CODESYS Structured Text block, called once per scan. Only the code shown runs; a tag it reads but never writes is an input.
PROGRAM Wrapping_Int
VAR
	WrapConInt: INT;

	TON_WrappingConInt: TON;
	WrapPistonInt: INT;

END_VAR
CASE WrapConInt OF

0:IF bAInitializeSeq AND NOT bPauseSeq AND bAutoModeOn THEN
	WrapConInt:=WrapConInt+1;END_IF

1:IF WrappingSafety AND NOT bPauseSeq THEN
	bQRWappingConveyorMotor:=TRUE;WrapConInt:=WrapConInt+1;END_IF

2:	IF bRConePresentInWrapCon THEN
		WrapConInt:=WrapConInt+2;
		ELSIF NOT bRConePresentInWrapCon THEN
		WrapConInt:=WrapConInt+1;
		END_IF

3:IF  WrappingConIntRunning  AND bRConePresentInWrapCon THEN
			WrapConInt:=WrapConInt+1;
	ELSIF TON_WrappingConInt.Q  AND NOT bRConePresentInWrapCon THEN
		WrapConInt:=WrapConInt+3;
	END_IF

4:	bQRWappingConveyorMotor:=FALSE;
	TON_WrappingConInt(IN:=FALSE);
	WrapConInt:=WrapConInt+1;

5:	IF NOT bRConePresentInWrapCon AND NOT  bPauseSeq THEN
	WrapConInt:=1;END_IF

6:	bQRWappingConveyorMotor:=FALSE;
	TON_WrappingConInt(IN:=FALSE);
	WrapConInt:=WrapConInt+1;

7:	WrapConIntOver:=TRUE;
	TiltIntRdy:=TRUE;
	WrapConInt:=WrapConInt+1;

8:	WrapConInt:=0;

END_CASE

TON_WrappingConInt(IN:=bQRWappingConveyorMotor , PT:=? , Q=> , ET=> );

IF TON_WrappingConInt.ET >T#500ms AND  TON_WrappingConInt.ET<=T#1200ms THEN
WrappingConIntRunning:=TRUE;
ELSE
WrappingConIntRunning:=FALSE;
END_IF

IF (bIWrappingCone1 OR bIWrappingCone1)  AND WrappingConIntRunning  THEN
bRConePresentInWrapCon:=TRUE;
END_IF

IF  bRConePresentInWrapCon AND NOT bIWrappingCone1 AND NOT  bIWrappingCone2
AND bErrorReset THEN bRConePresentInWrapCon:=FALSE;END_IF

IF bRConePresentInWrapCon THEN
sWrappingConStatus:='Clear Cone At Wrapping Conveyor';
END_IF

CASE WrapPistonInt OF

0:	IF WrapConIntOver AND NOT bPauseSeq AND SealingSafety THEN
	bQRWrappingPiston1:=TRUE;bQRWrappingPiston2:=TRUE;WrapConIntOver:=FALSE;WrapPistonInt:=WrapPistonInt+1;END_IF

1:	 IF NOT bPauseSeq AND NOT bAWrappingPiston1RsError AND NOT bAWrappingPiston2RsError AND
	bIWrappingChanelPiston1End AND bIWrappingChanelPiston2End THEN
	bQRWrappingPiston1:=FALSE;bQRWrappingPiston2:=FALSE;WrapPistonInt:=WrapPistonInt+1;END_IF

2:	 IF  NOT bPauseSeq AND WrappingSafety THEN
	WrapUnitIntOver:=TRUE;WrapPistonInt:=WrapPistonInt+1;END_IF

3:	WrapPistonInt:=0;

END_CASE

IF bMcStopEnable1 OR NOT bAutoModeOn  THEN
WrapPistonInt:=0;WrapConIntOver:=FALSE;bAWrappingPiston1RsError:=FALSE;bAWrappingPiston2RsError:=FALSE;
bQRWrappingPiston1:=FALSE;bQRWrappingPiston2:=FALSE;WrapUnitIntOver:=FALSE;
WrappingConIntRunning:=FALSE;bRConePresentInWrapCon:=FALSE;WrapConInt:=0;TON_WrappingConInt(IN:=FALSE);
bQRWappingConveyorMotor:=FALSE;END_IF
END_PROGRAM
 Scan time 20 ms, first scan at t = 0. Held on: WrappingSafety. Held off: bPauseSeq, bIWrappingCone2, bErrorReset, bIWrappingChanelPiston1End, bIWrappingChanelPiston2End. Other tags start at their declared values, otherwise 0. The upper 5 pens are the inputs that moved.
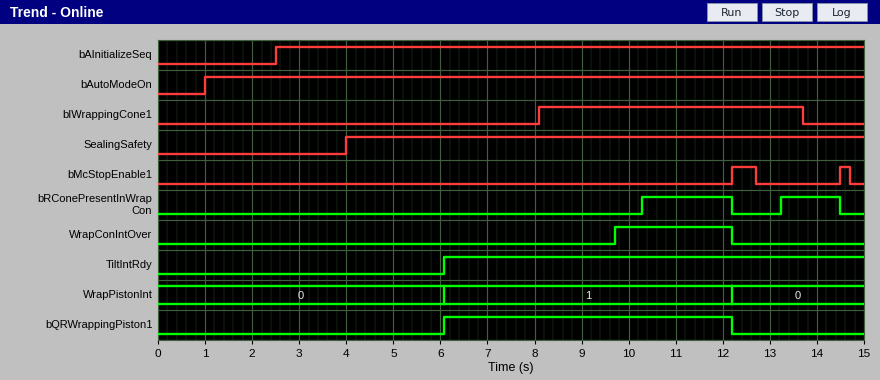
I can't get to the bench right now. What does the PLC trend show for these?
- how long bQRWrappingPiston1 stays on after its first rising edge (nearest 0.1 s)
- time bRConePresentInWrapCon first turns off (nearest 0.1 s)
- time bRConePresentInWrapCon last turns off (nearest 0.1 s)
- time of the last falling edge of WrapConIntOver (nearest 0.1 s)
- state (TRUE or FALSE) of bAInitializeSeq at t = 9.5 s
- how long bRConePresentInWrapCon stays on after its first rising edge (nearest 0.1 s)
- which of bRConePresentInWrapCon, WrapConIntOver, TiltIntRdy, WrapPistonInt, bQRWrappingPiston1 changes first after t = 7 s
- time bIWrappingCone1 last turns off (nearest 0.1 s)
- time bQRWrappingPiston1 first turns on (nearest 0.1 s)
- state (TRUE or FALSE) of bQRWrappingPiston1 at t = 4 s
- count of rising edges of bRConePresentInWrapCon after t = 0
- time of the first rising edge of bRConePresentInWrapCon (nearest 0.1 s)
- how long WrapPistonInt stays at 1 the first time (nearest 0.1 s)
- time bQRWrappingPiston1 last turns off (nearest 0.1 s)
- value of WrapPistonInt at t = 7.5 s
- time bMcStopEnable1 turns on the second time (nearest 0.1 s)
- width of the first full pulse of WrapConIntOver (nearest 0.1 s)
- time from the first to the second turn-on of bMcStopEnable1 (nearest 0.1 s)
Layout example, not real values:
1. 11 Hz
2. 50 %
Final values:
1. 6.1 s
2. 12.2 s
3. 14.5 s
4. 12.2 s
5. TRUE
6. 1.9 s
7. WrapConIntOver
8. 13.7 s
9. 6.1 s
10. FALSE
11. 2
12. 10.3 s
13. 6.1 s
14. 12.2 s
15. 1
16. 14.5 s
17. 2.5 s
18. 2.3 s
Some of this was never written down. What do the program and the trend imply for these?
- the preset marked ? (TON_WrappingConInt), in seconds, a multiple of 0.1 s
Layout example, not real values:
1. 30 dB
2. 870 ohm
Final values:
1. 3.5 s
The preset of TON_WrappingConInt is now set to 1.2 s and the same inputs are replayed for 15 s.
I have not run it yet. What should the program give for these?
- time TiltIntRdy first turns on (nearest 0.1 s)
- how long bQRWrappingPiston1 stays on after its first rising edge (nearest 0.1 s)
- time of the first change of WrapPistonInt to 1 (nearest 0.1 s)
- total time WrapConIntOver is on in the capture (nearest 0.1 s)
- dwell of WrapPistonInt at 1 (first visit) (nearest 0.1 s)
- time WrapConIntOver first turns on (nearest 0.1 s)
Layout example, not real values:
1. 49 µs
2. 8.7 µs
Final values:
1. 3.8 s
2. 8.2 s
3. 4.0 s
4. 7.3 s
5. 8.2 s
6. 3.8 s
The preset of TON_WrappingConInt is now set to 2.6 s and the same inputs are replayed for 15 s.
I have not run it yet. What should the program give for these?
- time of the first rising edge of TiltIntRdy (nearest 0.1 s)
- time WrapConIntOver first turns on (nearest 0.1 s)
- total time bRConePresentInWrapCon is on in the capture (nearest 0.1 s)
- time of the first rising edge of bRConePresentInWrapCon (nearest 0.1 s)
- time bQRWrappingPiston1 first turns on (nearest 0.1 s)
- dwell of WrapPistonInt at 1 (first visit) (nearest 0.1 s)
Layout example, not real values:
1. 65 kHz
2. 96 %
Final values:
1. 5.2 s
2. 7.9 s
3. 5.0 s
4. 8.5 s
5. 5.2 s
6. 7.0 s
